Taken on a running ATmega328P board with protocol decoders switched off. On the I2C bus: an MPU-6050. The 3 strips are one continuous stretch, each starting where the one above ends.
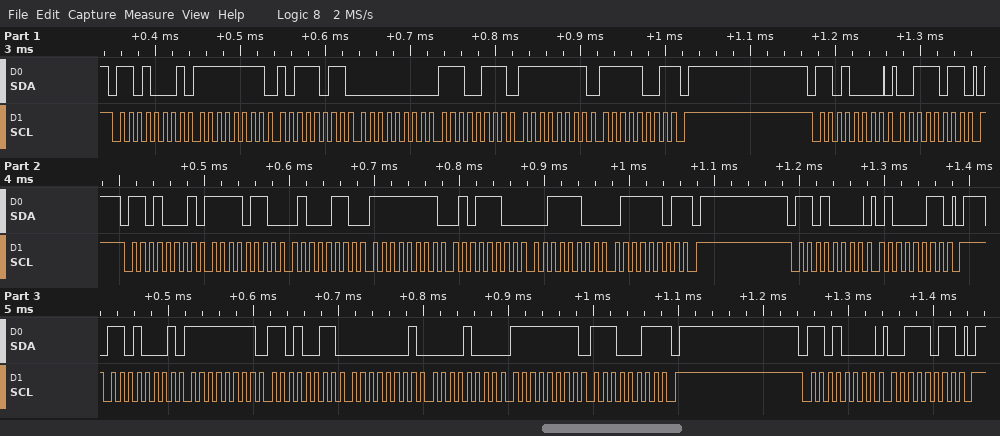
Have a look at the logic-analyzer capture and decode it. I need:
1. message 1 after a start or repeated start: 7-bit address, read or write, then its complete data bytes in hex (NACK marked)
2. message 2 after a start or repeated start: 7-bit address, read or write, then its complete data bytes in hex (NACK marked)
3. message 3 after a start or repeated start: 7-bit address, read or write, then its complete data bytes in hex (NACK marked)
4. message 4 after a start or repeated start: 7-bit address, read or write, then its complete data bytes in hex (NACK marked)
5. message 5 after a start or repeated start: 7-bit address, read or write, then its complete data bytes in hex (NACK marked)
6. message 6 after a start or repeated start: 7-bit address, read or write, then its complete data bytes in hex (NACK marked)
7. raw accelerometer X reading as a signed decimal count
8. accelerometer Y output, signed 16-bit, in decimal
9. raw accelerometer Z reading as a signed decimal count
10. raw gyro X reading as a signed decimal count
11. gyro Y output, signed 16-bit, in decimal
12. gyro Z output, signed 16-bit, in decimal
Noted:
0x68 read: FF BB 00 E7 FF F9 NACK
0x68 write: 3B
0x68 read: F6 46 FF 5C 3C 7D NACK
0x68 write: 43
0x68 read: FF D3 01 08 FF E3 NACK
0x68 write: 3B
-2490
-164
15485
-45
264
-29
